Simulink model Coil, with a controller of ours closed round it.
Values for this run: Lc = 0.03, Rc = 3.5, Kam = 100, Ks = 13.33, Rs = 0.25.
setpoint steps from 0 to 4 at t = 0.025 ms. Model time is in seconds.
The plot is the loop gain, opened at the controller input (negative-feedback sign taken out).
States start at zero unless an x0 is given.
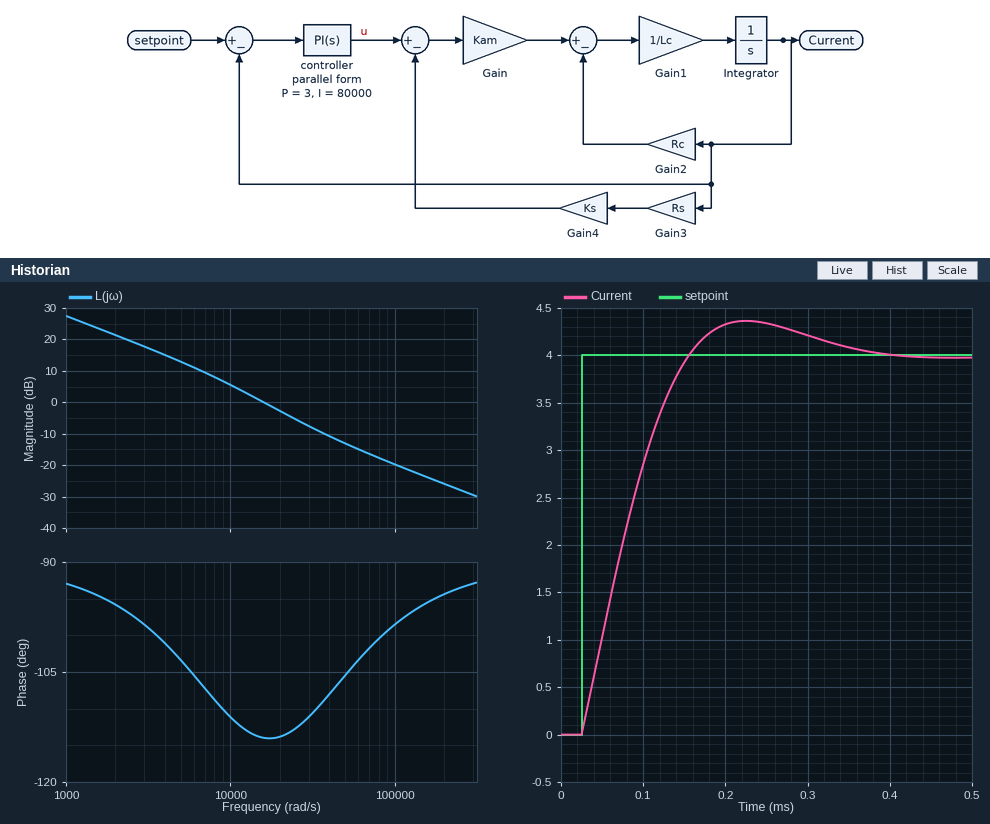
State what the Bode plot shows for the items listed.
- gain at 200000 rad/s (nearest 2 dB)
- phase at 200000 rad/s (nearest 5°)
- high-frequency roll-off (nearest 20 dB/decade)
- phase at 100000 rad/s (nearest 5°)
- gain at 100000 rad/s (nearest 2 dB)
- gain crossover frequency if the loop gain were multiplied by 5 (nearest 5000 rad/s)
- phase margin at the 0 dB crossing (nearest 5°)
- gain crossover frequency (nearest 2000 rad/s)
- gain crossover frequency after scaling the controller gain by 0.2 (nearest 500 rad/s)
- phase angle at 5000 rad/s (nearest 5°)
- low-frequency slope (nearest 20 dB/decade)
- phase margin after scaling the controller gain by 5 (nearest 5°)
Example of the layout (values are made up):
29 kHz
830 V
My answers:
-26 dB
-95°
-20 dB/decade
-100°
-20 dB
55000 rad/s
65°
16000 rad/s
4500 rad/s
-105°
-20 dB/decade
75°
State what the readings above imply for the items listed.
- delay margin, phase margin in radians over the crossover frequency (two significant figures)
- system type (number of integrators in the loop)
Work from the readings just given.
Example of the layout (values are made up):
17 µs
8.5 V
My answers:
0.000071 s
1
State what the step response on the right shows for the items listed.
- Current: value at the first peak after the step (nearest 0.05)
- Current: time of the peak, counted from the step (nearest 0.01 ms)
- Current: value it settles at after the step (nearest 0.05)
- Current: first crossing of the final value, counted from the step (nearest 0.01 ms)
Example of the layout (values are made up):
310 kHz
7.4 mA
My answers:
4.35
0.20 ms
4.00
0.13 ms
